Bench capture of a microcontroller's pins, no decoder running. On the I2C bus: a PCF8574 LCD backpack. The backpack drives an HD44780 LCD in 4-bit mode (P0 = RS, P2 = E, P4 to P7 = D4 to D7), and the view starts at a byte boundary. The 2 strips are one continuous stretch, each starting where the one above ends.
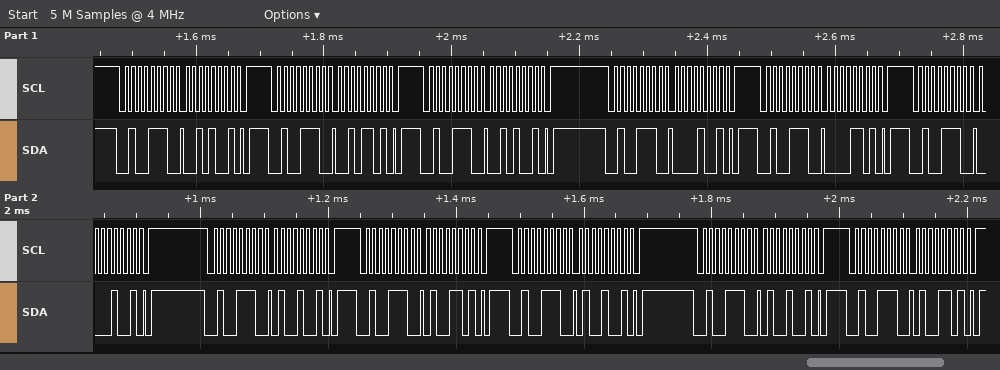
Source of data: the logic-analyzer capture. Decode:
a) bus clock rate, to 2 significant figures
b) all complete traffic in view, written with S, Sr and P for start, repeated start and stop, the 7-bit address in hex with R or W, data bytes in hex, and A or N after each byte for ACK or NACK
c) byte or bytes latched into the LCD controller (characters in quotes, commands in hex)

100 kHz
S 27W A 29 A P S 27W A 2D A P S 27W A 29 A P S 27W A 09 A P S 27W A 0D A P S 27W A 09 A P S 27W A 49 A P S 27W A 4D A P S 27W A 49 A P S 27W A 49 A P S 27W A 4D A P
' '
